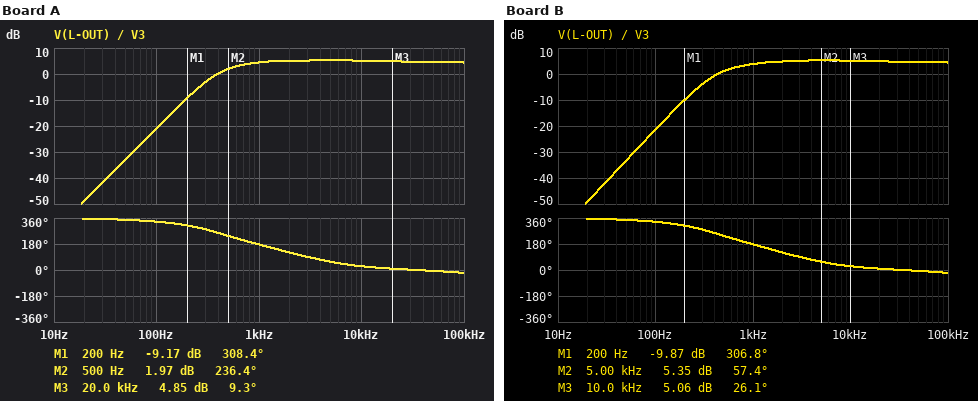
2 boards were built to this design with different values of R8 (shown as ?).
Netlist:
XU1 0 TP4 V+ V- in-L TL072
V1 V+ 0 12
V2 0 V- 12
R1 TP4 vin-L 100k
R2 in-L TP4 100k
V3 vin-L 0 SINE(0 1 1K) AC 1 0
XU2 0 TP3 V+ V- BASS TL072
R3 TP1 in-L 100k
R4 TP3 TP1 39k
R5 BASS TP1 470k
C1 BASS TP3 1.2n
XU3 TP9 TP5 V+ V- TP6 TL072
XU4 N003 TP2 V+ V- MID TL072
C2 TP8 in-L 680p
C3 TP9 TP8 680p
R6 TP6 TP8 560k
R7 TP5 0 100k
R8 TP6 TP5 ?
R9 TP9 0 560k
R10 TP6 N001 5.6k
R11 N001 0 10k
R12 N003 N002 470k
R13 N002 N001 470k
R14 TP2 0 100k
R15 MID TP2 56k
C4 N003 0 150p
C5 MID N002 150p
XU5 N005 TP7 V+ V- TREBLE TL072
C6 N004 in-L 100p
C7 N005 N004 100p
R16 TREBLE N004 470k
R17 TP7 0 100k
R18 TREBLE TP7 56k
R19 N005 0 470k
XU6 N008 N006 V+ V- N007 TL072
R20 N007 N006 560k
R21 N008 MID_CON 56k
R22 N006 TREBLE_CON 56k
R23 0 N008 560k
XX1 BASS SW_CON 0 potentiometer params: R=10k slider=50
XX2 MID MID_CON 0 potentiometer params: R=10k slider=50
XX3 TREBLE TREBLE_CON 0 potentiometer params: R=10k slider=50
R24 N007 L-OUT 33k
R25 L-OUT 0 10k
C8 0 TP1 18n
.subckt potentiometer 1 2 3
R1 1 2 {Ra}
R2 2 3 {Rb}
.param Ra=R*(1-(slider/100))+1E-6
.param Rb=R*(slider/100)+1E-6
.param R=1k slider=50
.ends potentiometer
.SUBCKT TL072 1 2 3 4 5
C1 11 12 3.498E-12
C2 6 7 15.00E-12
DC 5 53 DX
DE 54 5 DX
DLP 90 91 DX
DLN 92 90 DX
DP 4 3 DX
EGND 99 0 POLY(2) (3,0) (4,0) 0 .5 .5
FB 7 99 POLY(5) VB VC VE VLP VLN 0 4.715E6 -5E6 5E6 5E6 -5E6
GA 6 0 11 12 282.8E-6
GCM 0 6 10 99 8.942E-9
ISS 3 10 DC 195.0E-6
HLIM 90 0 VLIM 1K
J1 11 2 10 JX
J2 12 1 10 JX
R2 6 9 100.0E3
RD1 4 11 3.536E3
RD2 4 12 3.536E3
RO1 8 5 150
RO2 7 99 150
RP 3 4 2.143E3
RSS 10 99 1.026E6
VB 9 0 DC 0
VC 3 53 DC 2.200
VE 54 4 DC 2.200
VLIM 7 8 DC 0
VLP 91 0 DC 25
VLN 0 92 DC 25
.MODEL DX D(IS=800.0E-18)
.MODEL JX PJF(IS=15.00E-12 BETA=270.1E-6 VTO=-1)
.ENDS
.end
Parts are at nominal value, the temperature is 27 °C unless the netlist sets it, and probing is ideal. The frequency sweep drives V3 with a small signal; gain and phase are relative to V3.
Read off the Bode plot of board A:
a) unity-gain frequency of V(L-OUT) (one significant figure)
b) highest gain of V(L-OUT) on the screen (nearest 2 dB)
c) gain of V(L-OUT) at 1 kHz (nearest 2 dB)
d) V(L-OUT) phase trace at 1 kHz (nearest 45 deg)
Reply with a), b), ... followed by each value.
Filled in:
a) 400 Hz
b) 6 dB
c) 4 dB
d) 180 deg
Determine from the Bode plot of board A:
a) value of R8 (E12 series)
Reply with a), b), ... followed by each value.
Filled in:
a) 47 kΩ
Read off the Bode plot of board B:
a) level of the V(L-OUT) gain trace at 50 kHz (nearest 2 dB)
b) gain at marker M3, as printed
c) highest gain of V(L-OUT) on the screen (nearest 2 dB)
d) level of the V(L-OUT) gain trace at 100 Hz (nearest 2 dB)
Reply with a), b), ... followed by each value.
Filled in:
a) 4 dB
b) 5.06 dB
c) 6 dB
d) -22 dB
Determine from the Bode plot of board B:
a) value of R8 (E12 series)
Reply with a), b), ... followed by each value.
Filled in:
a) 39 kΩ
